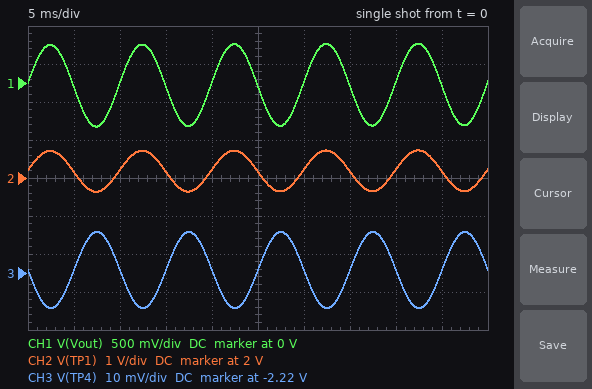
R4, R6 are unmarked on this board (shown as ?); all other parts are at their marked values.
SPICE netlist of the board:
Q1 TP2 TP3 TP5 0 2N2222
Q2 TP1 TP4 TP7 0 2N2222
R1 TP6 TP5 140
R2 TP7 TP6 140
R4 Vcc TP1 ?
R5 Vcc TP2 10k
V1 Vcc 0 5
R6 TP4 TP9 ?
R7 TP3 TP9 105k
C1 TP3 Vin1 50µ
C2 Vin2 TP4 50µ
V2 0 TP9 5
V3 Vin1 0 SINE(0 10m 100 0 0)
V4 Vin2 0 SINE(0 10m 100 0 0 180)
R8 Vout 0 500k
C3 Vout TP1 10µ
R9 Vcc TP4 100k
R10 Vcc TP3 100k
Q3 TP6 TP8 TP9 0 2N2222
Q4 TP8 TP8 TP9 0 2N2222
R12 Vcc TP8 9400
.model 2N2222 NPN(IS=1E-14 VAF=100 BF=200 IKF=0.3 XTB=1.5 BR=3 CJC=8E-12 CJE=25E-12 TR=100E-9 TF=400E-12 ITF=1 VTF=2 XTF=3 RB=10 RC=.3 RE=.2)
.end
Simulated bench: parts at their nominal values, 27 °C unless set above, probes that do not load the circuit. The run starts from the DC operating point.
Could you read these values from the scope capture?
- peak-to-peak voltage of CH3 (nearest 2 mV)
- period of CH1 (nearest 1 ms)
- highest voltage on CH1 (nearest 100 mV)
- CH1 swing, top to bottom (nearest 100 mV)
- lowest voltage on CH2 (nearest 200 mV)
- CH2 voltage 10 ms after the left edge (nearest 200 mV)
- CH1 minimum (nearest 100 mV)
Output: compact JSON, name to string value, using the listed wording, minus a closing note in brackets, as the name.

{"peak-to-peak voltage of CH3": "20 mV", "period of CH1": "10 ms", "highest voltage on CH1": "500 mV", "CH1 swing, top to bottom": "1.1 V", "lowest voltage on CH2": "1.6 V", "CH2 voltage 10 ms after the left edge": "2.2 V", "CH1 minimum": "-600 mV"}
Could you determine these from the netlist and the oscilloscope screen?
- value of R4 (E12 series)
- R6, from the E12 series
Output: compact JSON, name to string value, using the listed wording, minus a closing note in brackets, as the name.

{"value of R4": "15 kΩ", "R6, from the E12 series": "39 kΩ"}
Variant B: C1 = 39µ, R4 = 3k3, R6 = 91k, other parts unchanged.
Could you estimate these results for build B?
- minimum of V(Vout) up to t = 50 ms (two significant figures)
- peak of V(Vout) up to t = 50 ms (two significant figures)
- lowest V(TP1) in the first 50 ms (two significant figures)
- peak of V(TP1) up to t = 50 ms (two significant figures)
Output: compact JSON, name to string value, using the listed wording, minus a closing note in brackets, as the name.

{"minimum of V(Vout) up to t = 50 ms": "-220 mV", "peak of V(Vout) up to t = 50 ms": "120 mV", "lowest V(TP1) in the first 50 ms": "3.4 V", "peak of V(TP1) up to t = 50 ms": "3.7 V"}
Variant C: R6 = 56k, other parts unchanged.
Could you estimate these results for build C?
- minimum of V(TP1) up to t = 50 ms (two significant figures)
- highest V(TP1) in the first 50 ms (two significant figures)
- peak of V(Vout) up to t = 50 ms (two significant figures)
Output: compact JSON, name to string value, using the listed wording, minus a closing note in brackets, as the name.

{"minimum of V(TP1) up to t = 50 ms": "140 mV", "highest V(TP1) in the first 50 ms": "1.3 V", "peak of V(Vout) up to t = 50 ms": "540 mV"}
